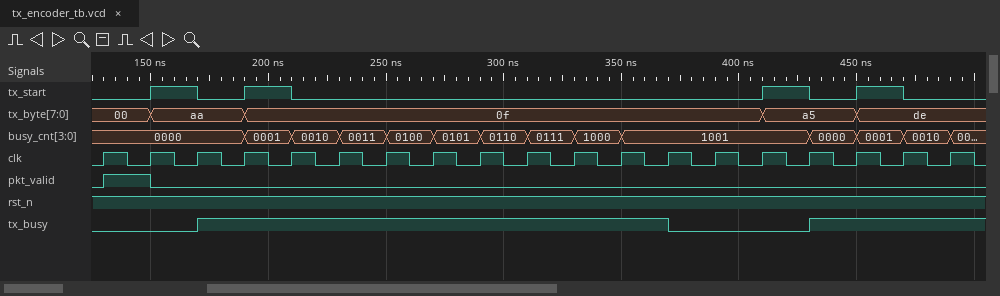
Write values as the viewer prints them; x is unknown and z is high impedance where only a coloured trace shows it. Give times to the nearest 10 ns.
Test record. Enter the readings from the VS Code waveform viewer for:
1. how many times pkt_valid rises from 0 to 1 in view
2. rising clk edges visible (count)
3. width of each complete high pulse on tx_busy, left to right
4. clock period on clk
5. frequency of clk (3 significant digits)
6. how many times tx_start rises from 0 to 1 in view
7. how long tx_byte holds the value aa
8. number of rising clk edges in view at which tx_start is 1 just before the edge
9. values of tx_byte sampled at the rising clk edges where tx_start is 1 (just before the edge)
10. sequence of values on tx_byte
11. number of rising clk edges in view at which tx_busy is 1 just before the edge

1
19
200 ns
20 ns
50.0 MHz
4
40 ns
4
aa, 0f, a5, de
00, aa, 0f, a5, de
13
